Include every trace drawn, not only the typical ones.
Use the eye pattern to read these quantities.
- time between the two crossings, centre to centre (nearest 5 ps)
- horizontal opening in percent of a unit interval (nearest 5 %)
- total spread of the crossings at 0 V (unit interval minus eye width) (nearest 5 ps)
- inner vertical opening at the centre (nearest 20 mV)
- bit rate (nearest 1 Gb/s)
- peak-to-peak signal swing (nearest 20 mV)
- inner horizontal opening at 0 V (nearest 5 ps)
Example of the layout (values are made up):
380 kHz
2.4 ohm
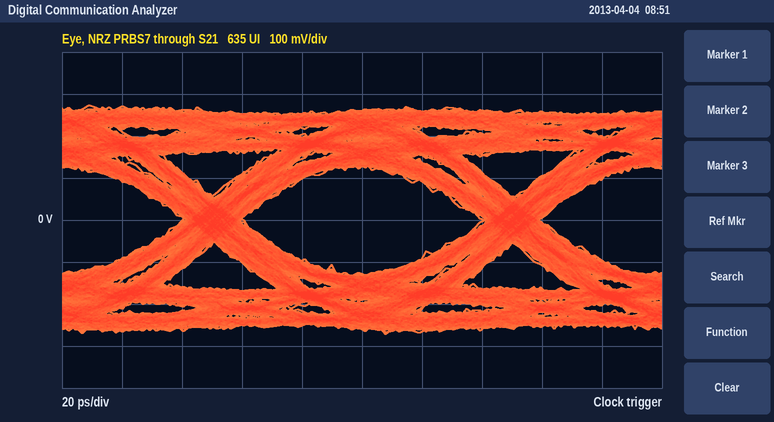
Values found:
100 ps
80 %
20 ps
260 mV
10 Gb/s
540 mV
80 ps
